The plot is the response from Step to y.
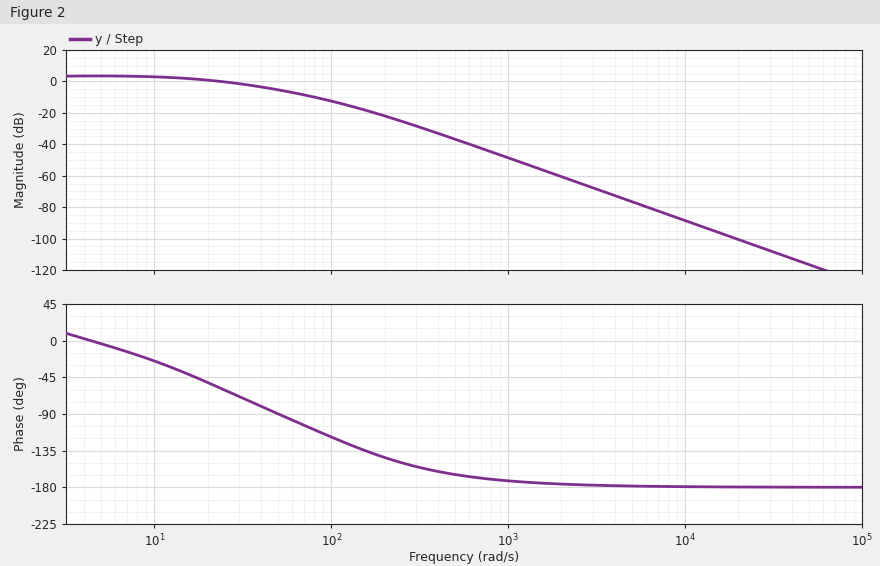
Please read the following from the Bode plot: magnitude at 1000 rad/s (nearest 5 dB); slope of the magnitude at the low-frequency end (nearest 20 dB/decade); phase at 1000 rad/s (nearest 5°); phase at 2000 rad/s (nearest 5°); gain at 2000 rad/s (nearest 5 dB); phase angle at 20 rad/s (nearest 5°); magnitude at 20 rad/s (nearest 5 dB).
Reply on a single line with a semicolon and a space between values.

-50 dB; 0 dB/decade; -170°; -175°; -60 dB; -50°; 0 dB
